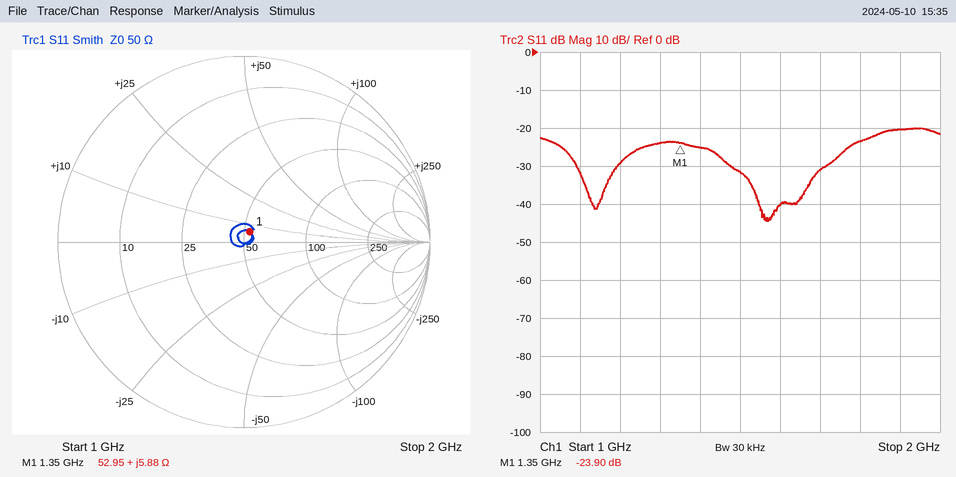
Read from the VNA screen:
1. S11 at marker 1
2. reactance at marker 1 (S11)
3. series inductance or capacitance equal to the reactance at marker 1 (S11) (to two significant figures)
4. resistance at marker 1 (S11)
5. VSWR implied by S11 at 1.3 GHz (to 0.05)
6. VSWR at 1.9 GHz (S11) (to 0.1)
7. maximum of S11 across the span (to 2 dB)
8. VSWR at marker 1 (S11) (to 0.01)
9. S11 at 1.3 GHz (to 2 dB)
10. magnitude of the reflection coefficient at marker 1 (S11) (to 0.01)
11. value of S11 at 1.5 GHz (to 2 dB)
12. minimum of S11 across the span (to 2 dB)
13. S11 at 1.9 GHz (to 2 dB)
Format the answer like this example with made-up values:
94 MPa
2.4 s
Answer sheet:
-23.90 dB
+5.88 Ω
690 pH
52.95 Ω
1.15
1.2
-20 dB
1.14
-24 dB
0.06
-32 dB
-44 dB
-20 dB
